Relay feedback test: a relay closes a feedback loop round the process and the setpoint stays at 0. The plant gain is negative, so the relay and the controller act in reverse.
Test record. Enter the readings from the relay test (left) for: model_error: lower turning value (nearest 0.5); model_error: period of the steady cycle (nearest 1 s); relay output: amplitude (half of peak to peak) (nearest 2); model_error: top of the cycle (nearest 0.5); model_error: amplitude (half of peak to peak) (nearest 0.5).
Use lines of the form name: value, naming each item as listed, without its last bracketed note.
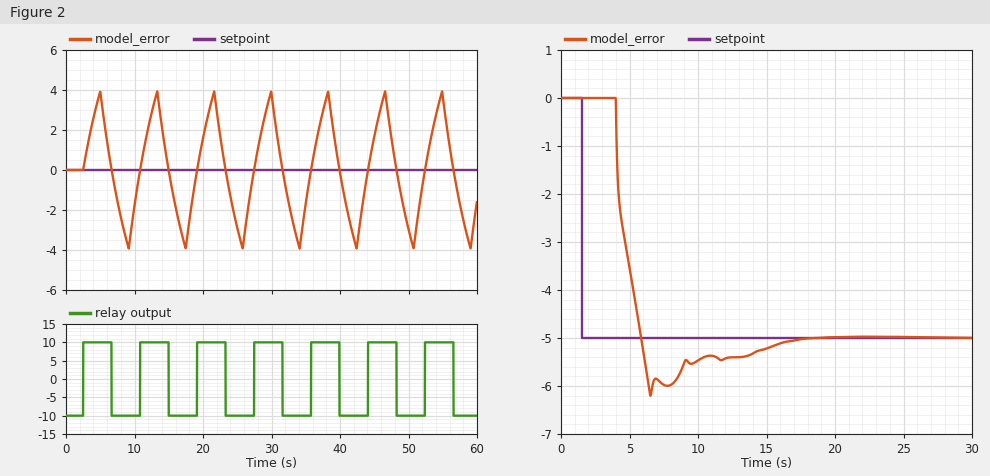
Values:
model_error: lower turning value: -4.0
model_error: period of the steady cycle: 8 s
relay output: amplitude (half of peak to peak): 10
model_error: top of the cycle: 4.0
model_error: amplitude (half of peak to peak): 4.0
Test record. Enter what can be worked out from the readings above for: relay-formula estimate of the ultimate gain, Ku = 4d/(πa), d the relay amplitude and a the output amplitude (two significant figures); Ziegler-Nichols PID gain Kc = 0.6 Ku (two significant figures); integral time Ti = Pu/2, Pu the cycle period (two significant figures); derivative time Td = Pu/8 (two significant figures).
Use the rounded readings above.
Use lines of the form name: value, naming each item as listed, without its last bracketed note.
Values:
relay-formula estimate of the ultimate gain, Ku = 4d/(πa), d the relay amplitude and a the output amplitude: 3.2
Ziegler-Nichols PID gain Kc = 0.6 Ku: 1.9
integral time Ti = Pu/2, Pu the cycle period: 4.0 s
derivative time Td = Pu/8: 1.0 s
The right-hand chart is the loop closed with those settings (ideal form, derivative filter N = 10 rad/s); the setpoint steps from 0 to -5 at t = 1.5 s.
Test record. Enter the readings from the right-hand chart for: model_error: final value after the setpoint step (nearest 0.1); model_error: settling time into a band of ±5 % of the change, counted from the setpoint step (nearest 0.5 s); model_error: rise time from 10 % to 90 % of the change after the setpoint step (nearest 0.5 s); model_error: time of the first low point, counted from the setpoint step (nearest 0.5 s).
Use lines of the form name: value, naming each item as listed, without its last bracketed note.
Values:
model_error: final value after the setpoint step: -5.0
model_error: settling time into a band of ±5 % of the change, counted from the setpoint step: 13.0 s
model_error: rise time from 10 % to 90 % of the change after the setpoint step: 1.5 s
model_error: time of the first low point, counted from the setpoint step: 5.0 s
